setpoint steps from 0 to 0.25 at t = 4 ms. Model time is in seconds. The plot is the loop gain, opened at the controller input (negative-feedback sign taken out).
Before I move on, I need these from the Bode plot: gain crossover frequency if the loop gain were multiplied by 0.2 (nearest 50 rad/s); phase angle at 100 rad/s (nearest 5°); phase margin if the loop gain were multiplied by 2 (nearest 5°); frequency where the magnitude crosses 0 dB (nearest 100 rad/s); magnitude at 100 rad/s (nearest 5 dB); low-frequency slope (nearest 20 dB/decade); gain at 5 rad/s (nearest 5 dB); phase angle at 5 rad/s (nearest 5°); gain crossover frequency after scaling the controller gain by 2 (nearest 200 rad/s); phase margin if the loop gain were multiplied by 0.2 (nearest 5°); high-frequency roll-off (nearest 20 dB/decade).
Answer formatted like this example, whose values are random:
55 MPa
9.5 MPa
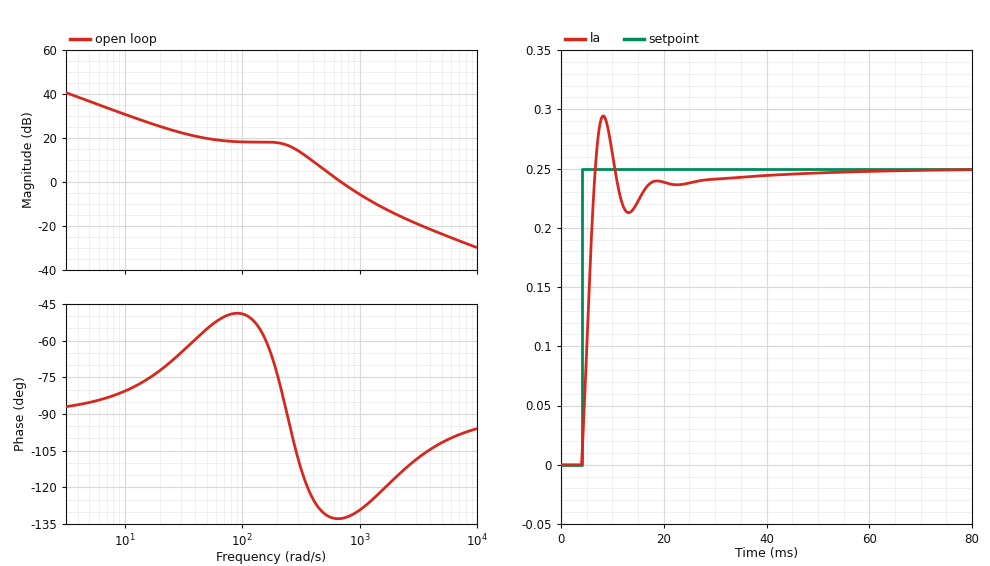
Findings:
300 rad/s
-50°
50°
700 rad/s
20 dB
-20 dB/decade
35 dB
-85°
1000 rad/s
70°
-20 dB/decade
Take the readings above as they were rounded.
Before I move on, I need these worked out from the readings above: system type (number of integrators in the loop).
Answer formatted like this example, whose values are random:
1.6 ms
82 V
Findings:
1
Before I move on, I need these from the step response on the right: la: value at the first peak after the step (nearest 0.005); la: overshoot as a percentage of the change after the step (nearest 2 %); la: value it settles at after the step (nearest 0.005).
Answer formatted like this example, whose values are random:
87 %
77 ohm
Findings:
0.295
18 %
0.250
